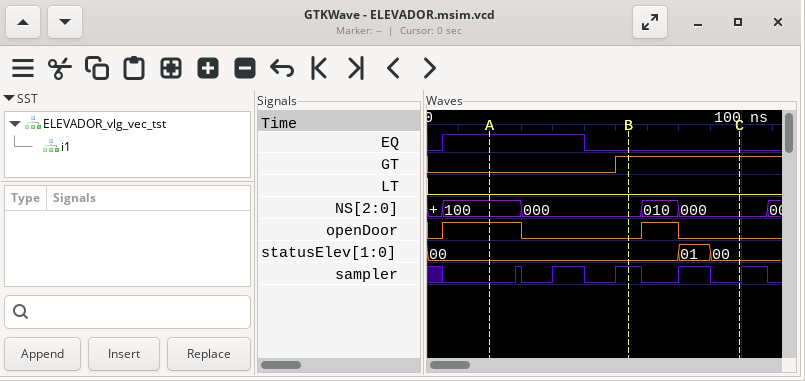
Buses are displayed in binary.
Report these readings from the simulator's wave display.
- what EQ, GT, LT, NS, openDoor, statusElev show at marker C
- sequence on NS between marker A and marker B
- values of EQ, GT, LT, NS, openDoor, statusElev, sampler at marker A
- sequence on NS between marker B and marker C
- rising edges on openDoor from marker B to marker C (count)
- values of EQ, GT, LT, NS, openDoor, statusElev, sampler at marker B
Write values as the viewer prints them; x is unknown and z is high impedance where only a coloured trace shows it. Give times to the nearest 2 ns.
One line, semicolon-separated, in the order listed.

EQ=0, GT=1, LT=0, NS=000, openDoor=0, statusElev=00; 100, 000; EQ=1, GT=0, LT=0, NS=100, openDoor=1, statusElev=00, sampler=0; 000, 010, 000; 1; EQ=0, GT=1, LT=0, NS=000, openDoor=0, statusElev=00, sampler=1
